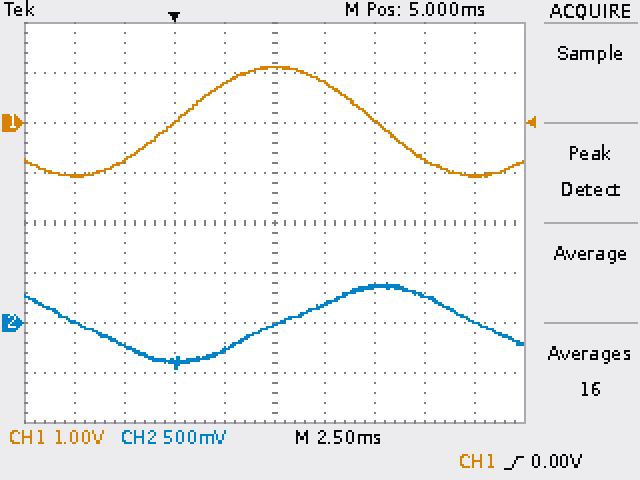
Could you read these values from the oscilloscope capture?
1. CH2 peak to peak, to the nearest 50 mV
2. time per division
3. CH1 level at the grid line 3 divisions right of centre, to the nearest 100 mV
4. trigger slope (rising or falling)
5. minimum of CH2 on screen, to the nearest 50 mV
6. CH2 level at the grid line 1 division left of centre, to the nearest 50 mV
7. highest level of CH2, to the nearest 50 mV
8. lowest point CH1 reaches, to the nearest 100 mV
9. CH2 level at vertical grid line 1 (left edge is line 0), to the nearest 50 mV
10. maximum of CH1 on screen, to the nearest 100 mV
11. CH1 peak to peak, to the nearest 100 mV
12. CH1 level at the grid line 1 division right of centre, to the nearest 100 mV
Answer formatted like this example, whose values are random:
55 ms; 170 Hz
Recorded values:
850 mV; 2.5 ms; -700 mV; rising; -450 mV; -250 mV; 400 mV; -1.1 V; 0 mV; 1.1 V; 2.2 V; 800 mV
